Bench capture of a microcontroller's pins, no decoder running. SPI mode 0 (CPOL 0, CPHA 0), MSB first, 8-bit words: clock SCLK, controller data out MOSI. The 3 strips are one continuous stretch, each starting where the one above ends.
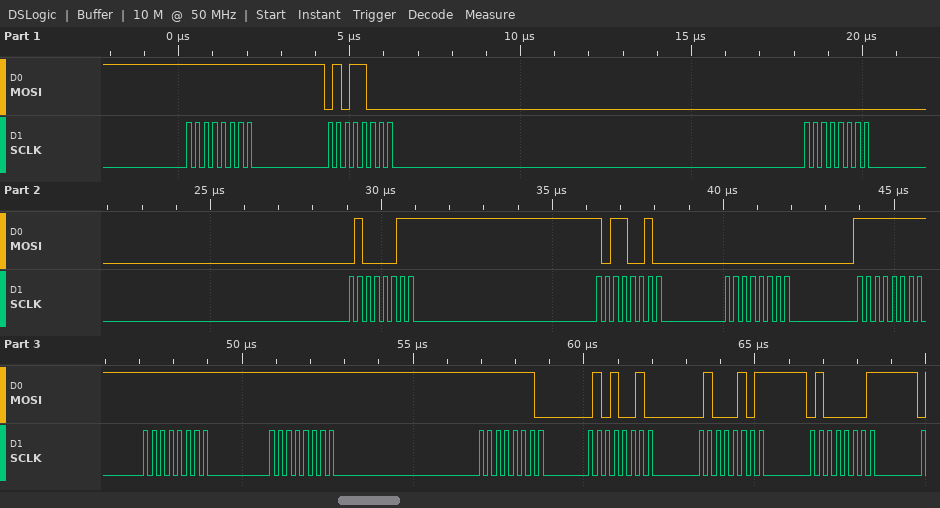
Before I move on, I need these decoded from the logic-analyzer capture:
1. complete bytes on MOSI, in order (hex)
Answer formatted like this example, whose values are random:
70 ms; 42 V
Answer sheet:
FF 58 00 43 B2 00 FF FF FF FE 52 45 41
